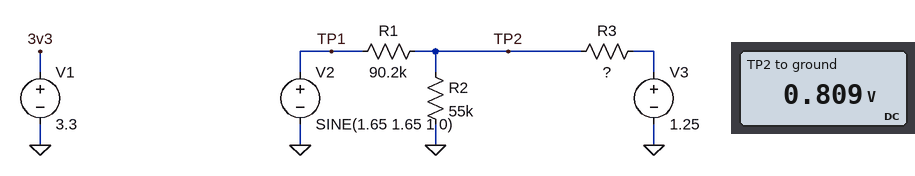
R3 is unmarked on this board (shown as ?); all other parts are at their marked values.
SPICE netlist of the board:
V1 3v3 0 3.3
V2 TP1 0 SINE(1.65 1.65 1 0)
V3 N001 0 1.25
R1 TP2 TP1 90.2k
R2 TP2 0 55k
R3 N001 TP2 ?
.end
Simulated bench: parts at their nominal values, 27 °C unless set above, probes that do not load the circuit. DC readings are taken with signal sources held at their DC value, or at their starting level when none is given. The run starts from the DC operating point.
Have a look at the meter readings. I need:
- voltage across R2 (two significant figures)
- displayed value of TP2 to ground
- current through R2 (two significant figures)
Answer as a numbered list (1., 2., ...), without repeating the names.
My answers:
1. 810 mV
2. 0.809 V
3. 15 µA
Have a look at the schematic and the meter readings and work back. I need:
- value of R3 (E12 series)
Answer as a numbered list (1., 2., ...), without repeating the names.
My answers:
1. 82 kΩ
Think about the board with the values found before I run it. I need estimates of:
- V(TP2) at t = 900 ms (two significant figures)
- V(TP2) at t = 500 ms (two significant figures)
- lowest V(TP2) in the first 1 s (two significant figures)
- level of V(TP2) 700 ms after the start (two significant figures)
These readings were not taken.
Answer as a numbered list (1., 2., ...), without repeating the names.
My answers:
1. 550 mV
2. 810 mV
3. 370 mV
4. 390 mV
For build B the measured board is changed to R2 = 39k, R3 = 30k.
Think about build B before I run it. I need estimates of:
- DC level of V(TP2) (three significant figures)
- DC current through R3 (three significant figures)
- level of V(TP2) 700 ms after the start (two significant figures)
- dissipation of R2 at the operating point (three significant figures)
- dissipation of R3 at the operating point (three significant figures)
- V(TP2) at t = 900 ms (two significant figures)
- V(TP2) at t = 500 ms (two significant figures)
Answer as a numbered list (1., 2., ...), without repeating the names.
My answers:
1. 856 mV
2. 13.1 µA
3. 610 mV
4. 18.8 µW
5. 5.18 µW
6. 700 mV
7. 860 mV
